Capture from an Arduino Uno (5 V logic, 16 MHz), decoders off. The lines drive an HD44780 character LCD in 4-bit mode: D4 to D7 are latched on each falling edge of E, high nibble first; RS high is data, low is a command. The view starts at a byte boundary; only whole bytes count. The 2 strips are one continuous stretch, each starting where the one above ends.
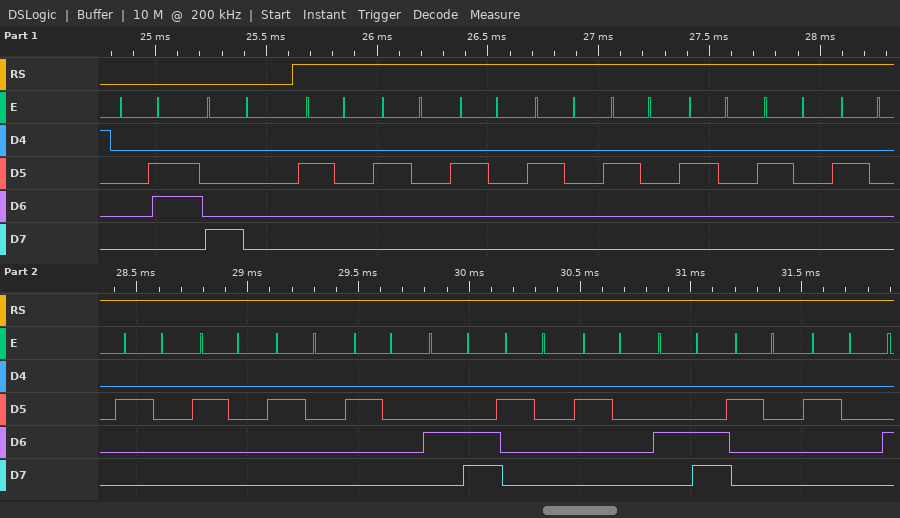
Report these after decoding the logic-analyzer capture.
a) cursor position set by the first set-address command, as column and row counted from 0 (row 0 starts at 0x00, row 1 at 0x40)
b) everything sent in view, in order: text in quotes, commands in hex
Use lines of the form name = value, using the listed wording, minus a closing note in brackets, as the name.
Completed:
cursor position set by the first set-address command, as column and row counted from 0 = column 0, row 0
everything sent in view, in order: text in quotes, commands in hex = 0x06 0x80 "            L  L  "
